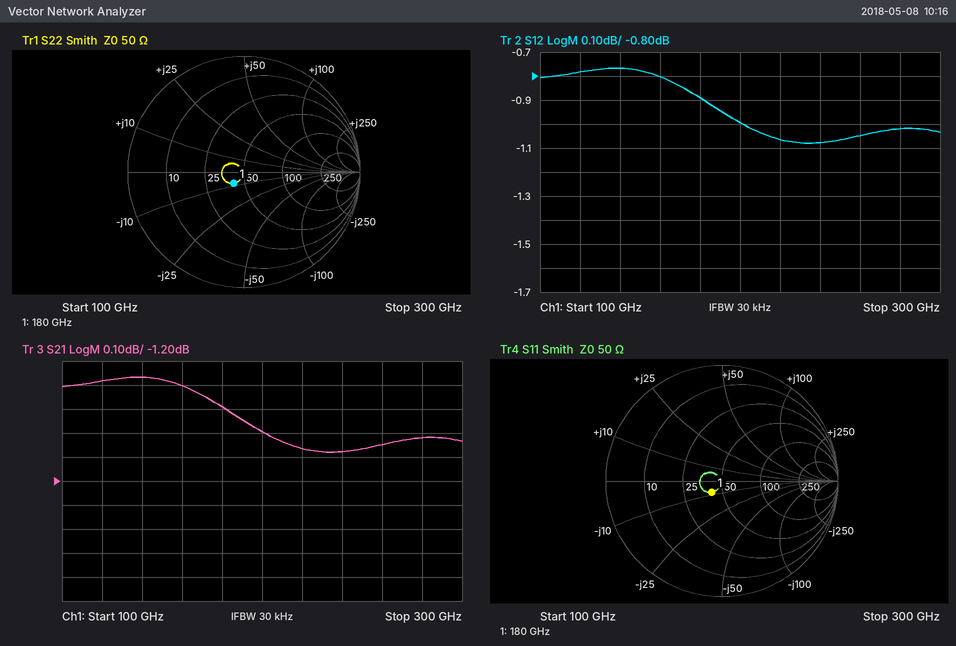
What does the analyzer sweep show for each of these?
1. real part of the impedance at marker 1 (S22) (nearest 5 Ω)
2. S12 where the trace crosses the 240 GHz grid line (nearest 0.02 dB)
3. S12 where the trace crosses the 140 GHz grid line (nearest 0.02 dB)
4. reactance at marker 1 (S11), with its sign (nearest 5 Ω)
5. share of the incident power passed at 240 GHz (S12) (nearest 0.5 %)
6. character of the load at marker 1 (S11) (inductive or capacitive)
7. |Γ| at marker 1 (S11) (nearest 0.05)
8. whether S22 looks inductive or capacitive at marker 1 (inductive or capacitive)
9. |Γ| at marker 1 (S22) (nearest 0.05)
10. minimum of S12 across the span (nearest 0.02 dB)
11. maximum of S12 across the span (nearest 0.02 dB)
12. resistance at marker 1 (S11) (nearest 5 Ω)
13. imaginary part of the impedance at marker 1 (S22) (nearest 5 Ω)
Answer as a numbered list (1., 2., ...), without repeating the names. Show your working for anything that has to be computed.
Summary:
1. 40 Ω
2. -1.08 dB
3. -0.76 dB
4. -10 Ω
5. 10^(-1.08/10) ≈ 78.0 %
6. capacitive
7. 0.15
8. capacitive
9. 0.15
10. -1.08 dB
11. -0.76 dB
12. 40 Ω
13. -10 Ω
